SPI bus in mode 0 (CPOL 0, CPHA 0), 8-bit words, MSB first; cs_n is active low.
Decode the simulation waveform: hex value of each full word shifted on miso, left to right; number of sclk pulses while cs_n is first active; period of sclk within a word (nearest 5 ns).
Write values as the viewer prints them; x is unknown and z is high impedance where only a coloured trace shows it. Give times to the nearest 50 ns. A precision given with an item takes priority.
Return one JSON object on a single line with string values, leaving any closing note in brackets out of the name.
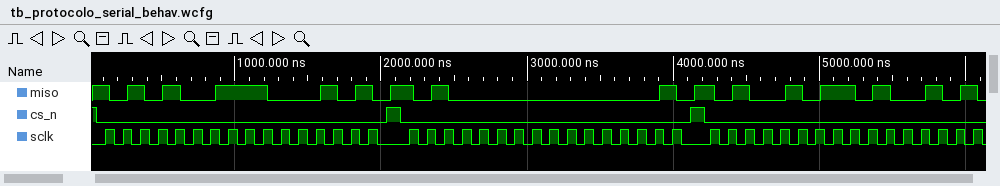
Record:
{"hex value of each full word shifted on miso, left to right": "A9, C5, A0, 01, A5, A5", "number of sclk pulses while cs_n is first active": "16", "period of sclk within a word": "120 ns"}
